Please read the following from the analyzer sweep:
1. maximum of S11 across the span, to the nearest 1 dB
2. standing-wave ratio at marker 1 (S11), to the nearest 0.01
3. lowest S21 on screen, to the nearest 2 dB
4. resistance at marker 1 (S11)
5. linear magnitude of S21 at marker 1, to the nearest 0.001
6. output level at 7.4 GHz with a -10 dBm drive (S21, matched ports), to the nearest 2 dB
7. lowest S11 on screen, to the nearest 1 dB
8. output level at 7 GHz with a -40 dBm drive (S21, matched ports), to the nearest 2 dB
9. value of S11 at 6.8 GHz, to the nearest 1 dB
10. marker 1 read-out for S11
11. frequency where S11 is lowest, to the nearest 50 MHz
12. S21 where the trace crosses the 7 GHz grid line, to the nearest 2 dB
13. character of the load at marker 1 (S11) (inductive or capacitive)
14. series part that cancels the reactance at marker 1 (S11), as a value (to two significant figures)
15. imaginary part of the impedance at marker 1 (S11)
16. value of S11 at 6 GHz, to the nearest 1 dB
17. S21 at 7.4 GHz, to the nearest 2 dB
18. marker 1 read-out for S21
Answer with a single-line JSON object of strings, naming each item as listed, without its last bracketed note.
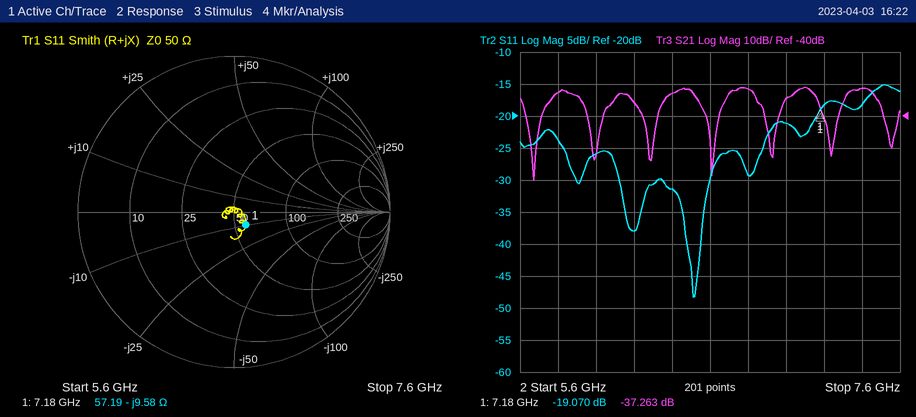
{"maximum of S11 across the span, to the nearest 1 dB": "-15 dB", "standing-wave ratio at marker 1 (S11), to the nearest 0.01": "1.25", "lowest S21 on screen, to the nearest 2 dB": "-60 dB", "resistance at marker 1": "57.19 Ω", "linear magnitude of S21 at marker 1, to the nearest 0.001": "0.014", "output level at 7.4 GHz with a -10 dBm drive (S21, matched ports), to the nearest 2 dB": "-42 dBm", "lowest S11 on screen, to the nearest 1 dB": "-48 dB", "output level at 7 GHz with a -40 dBm drive (S21, matched ports), to the nearest 2 dB": "-74 dBm", "value of S11 at 6.8 GHz, to the nearest 1 dB": "-29 dB", "marker 1 read-out for S11": "-19.070 dB", "frequency where S11 is lowest, to the nearest 50 MHz": "6.50 GHz", "S21 where the trace crosses the 7 GHz grid line, to the nearest 2 dB": "-34 dB", "character of the load at marker 1 (S11)": "capacitive", "series part that cancels the reactance at marker 1 (S11), as a value": "210 pH", "imaginary part of the impedance at marker 1": "-9.58 Ω", "value of S11 at 6 GHz, to the nearest 1 dB": "-26 dB", "S21 at 7.4 GHz, to the nearest 2 dB": "-32 dB", "marker 1 read-out for S21": "-37.263 dB"}
